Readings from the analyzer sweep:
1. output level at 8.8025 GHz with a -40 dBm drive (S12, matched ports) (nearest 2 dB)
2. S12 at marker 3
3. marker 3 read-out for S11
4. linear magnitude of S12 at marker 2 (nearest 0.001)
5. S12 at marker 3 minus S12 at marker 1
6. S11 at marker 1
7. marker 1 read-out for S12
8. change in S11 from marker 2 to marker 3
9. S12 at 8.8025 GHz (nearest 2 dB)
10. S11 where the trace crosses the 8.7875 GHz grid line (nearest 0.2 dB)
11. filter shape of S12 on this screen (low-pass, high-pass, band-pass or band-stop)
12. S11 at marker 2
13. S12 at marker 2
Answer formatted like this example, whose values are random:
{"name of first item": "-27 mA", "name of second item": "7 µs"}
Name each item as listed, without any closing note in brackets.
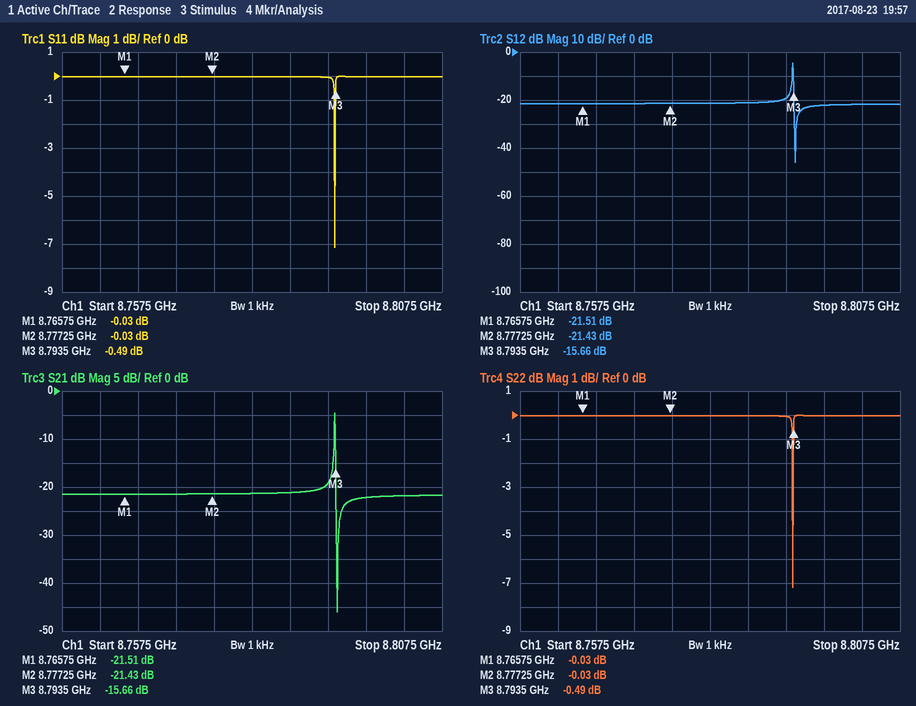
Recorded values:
{"output level at 8.8025 GHz with a -40 dBm drive (S12, matched ports)": "-62 dBm", "S12 at marker 3": "-15.66 dB", "marker 3 read-out for S11": "-0.49 dB", "linear magnitude of S12 at marker 2": "0.085", "S12 at marker 3 minus S12 at marker 1": "5.85 dB", "S11 at marker 1": "-0.03 dB", "marker 1 read-out for S12": "-21.51 dB", "change in S11 from marker 2 to marker 3": "-0.46 dB", "S12 at 8.8025 GHz": "-22 dB", "S11 where the trace crosses the 8.7875 GHz grid line": "0.0 dB", "filter shape of S12 on this screen": "band-pass", "S11 at marker 2": "-0.03 dB", "S12 at marker 2": "-21.43 dB"}
